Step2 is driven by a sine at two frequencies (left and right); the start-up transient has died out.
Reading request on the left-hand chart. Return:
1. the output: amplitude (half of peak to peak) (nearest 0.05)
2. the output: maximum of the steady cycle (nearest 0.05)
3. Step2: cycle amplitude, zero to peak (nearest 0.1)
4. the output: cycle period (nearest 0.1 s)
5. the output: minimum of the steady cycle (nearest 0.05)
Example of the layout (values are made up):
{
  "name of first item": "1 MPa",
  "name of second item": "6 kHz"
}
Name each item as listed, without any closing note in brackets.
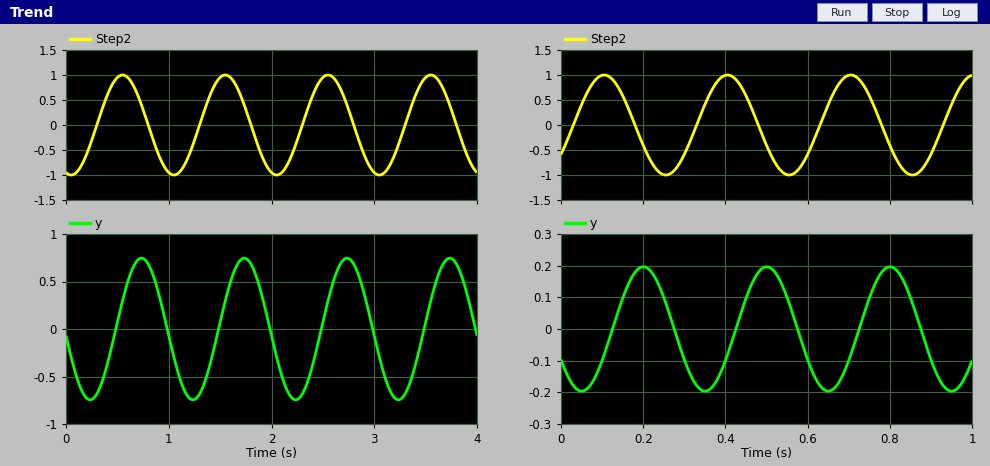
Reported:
{
  "the output: amplitude (half of peak to peak)": "0.75",
  "the output: maximum of the steady cycle": "0.75",
  "Step2: cycle amplitude, zero to peak": "1.0",
  "the output: cycle period": "1.0 s",
  "the output: minimum of the steady cycle": "-0.75"
}
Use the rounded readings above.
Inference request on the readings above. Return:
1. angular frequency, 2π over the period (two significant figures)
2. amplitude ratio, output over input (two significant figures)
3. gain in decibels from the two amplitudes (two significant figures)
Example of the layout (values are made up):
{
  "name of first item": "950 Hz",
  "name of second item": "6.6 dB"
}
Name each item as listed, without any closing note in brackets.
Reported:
{
  "angular frequency, 2π over the period": "6.3 rad/s",
  "amplitude ratio, output over input": "0.75",
  "gain in decibels from the two amplitudes": "-2.5 dB"
}
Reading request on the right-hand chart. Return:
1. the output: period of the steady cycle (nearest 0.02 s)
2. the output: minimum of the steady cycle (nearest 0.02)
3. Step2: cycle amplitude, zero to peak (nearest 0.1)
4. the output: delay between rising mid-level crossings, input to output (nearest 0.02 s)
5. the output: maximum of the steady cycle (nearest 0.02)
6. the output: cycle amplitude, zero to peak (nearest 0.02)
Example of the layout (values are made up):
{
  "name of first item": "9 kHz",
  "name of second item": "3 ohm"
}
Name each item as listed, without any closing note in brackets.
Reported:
{
  "the output: period of the steady cycle": "0.30 s",
  "the output: minimum of the steady cycle": "-0.20",
  "Step2: cycle amplitude, zero to peak": "1.0",
  "the output: delay between rising mid-level crossings, input to output": "0.10 s",
  "the output: maximum of the steady cycle": "0.20",
  "the output: cycle amplitude, zero to peak": "0.20"
}
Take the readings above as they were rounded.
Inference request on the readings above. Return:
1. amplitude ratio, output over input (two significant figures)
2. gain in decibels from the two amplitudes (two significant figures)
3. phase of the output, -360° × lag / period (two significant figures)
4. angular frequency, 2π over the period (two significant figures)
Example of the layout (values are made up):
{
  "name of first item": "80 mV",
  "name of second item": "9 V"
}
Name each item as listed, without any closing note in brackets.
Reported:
{
  "amplitude ratio, output over input": "0.20",
  "gain in decibels from the two amplitudes": "-14 dB",
  "phase of the output, -360° × lag / period": "-120°",
  "angular frequency, 2π over the period": "21 rad/s"
}
